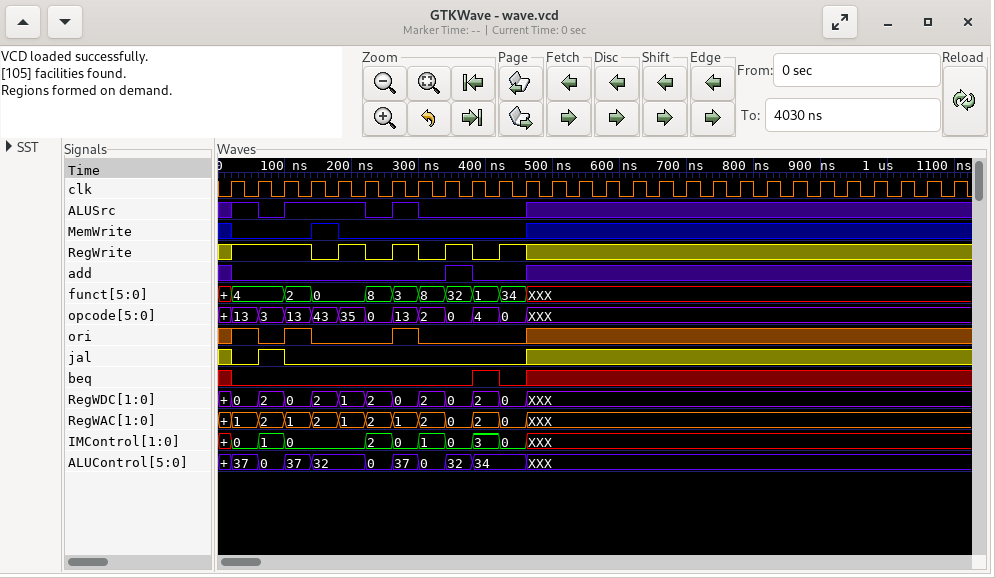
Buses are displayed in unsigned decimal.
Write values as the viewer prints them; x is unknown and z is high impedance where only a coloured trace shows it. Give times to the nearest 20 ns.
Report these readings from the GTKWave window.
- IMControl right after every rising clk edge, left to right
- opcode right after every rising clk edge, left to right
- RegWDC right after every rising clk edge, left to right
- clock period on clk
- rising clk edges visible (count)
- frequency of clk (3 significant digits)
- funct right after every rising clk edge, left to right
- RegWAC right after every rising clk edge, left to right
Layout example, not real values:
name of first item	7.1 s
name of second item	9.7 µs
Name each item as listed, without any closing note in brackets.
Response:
IMControl right after every rising clk edge, left to right	0, 1, 0, 0, 0, 2, 0, 1, 0, 3, 0, XXX, XXX, XXX, XXX, XXX, XXX, XXX, XXX, XXX, XXX, XXX, XXX, XXX, XXX, XXX, XXX, XXX
opcode right after every rising clk edge, left to right	13, 3, 13, 43, 35, 0, 13, 2, 0, 4, 0, XXX, XXX, XXX, XXX, XXX, XXX, XXX, XXX, XXX, XXX, XXX, XXX, XXX, XXX, XXX, XXX, XXX
RegWDC right after every rising clk edge, left to right	0, 2, 0, 2, 1, 2, 0, 2, 0, 2, 0, XXX, XXX, XXX, XXX, XXX, XXX, XXX, XXX, XXX, XXX, XXX, XXX, XXX, XXX, XXX, XXX, XXX
clock period on clk	40 ns
rising clk edges visible	28
frequency of clk	25.0 MHz
funct right after every rising clk edge, left to right	4, 4, 2, 0, 0, 8, 3, 8, 32, 1, 34, XXX, XXX, XXX, XXX, XXX, XXX, XXX, XXX, XXX, XXX, XXX, XXX, XXX, XXX, XXX, XXX, XXX
RegWAC right after every rising clk edge, left to right	1, 2, 1, 2, 1, 2, 1, 2, 0, 2, 0, XXX, XXX, XXX, XXX, XXX, XXX, XXX, XXX, XXX, XXX, XXX, XXX, XXX, XXX, XXX, XXX, XXX
